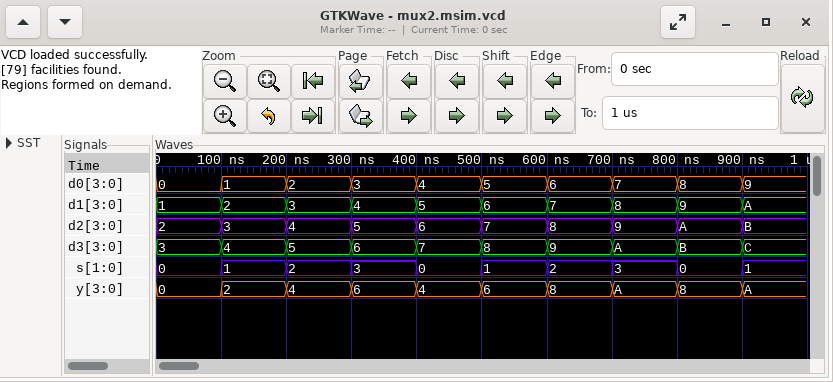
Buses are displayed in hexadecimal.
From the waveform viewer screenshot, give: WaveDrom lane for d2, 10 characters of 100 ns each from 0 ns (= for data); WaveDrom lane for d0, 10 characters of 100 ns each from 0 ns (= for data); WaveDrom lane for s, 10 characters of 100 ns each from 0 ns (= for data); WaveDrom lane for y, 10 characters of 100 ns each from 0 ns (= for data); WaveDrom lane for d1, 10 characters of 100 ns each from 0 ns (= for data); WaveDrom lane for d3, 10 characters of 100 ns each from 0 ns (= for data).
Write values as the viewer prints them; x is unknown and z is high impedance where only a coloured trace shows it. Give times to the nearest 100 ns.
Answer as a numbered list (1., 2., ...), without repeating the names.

1. {name: 'd2', wave: '==========', data: '2 3 4 5 6 7 8 9 A B'}
2. {name: 'd0', wave: '==========', data: '0 1 2 3 4 5 6 7 8 9'}
3. {name: 's', wave: '==========', data: '0 1 2 3 0 1 2 3 0 1'}
4. {name: 'y', wave: '==========', data: '0 2 4 6 4 6 8 A 8 A'}
5. {name: 'd1', wave: '==========', data: '1 2 3 4 5 6 7 8 9 A'}
6. {name: 'd3', wave: '==========', data: '3 4 5 6 7 8 9 A B C'}
